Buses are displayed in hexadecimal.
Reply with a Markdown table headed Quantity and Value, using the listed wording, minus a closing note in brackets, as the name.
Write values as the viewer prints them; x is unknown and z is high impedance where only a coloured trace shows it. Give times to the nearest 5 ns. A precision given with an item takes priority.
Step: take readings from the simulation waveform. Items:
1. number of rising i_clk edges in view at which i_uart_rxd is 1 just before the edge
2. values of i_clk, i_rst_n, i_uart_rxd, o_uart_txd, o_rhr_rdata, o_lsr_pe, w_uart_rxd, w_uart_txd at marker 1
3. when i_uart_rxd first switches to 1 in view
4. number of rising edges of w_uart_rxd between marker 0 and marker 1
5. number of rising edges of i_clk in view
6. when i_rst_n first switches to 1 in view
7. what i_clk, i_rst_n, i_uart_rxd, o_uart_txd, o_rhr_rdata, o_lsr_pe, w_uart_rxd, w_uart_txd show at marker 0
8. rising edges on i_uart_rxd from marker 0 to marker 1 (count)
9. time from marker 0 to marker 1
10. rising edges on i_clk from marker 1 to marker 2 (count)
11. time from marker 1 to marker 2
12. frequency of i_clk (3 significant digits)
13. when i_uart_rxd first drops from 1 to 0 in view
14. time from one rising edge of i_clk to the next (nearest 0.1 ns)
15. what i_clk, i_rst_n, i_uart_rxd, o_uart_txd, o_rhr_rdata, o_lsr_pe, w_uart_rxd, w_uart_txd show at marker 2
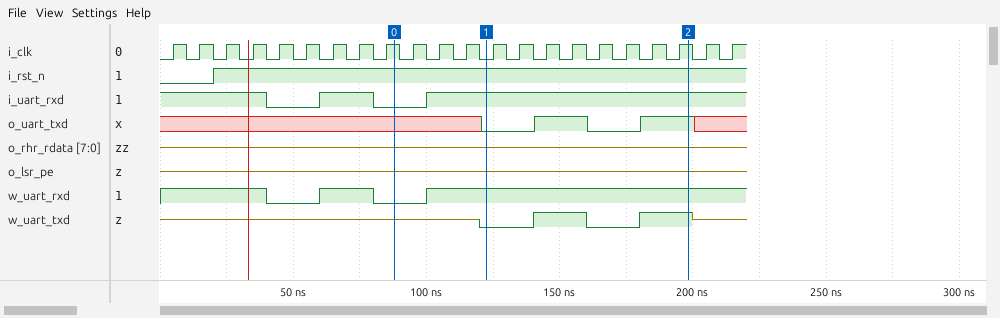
| Quantity | Value |
|---|---|
| number of rising i_clk edges in view at which i_uart_rxd is 1 just before the edge | 18 |
| values of i_clk, i_rst_n, i_uart_rxd, o_uart_txd, o_rhr_rdata, o_lsr_pe, w_uart_rxd, w_uart_txd at marker 1 | i_clk=0, i_rst_n=1, i_uart_rxd=1, o_uart_txd=0, o_rhr_rdata=z, o_lsr_pe=z, w_uart_rxd=1, w_uart_txd=0 |
| when i_uart_rxd first switches to 1 in view | 60 ns |
| number of rising edges of w_uart_rxd between marker 0 and marker 1 | 1 |
| number of rising edges of i_clk in view | 22 |
| when i_rst_n first switches to 1 in view | 20 ns |
| what i_clk, i_rst_n, i_uart_rxd, o_uart_txd, o_rhr_rdata, o_lsr_pe, w_uart_rxd, w_uart_txd show at marker 0 | i_clk=1, i_rst_n=1, i_uart_rxd=0, o_uart_txd=x, o_rhr_rdata=z, o_lsr_pe=z, w_uart_rxd=0, w_uart_txd=z |
| rising edges on i_uart_rxd from marker 0 to marker 1 | 1 |
| time from marker 0 to marker 1 | 35 ns |
| rising edges on i_clk from marker 1 to marker 2 | 8 |
| time from marker 1 to marker 2 | 75 ns |
| frequency of i_clk | 100 MHz |
| when i_uart_rxd first drops from 1 to 0 in view | 40 ns |
| time from one rising edge of i_clk to the next | 10 ns |
| what i_clk, i_rst_n, i_uart_rxd, o_uart_txd, o_rhr_rdata, o_lsr_pe, w_uart_rxd, w_uart_txd show at marker 2 | i_clk=1, i_rst_n=1, i_uart_rxd=1, o_uart_txd=1, o_rhr_rdata=z, o_lsr_pe=z, w_uart_rxd=1, w_uart_txd=1 |
